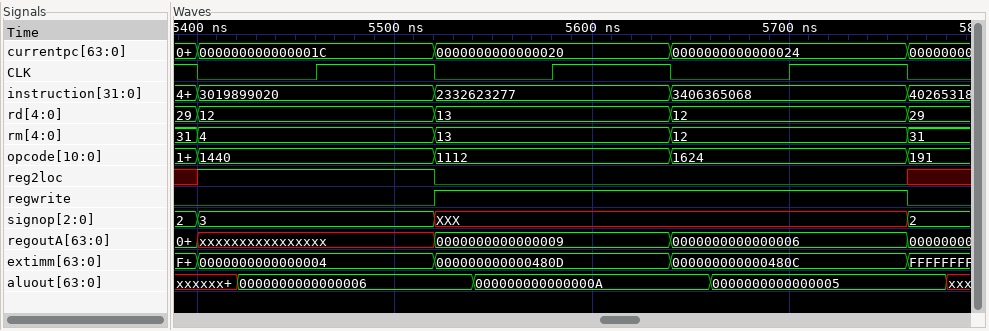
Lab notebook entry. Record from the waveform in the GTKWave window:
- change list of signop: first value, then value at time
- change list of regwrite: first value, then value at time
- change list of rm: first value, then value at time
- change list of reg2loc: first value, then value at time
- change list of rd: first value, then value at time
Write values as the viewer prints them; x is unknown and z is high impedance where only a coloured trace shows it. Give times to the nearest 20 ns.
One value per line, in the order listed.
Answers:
2, 3 at 5400 ns, XXX at 5520 ns, 2 at 5760 ns
0, 1 at 5520 ns, 0 at 5760 ns
31, 4 at 5400 ns, 13 at 5520 ns, 12 at 5640 ns, 31 at 5760 ns
x, 1 at 5400 ns, 0 at 5520 ns, x at 5760 ns
29, 12 at 5400 ns, 13 at 5520 ns, 12 at 5640 ns, 29 at 5760 ns
